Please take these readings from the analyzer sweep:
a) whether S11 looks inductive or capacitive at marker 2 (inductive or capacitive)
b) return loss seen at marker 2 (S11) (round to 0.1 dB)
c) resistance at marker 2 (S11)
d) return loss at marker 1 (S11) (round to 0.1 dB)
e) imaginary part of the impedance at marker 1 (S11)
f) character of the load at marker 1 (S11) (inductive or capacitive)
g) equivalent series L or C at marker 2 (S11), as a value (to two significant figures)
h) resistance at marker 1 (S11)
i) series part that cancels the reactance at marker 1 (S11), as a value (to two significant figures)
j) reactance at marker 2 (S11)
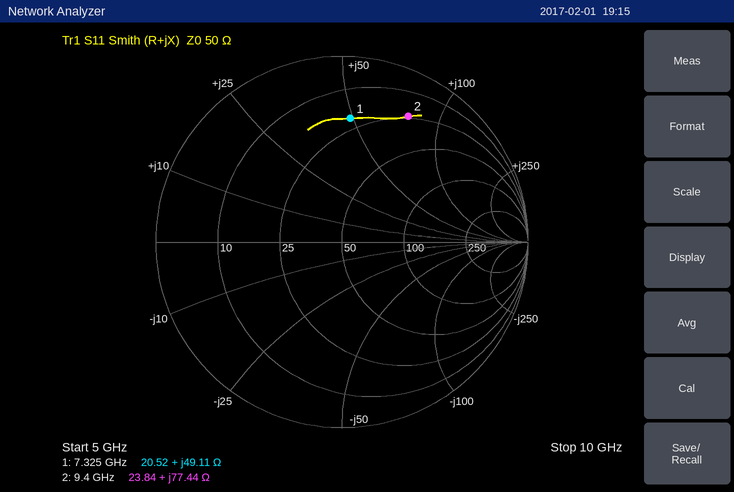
inductive
2.3 dB
23.84 Ω
3.5 dB
+49.11 Ω
inductive
1.3 nH
20.52 Ω
440 fF
+77.44 Ω
